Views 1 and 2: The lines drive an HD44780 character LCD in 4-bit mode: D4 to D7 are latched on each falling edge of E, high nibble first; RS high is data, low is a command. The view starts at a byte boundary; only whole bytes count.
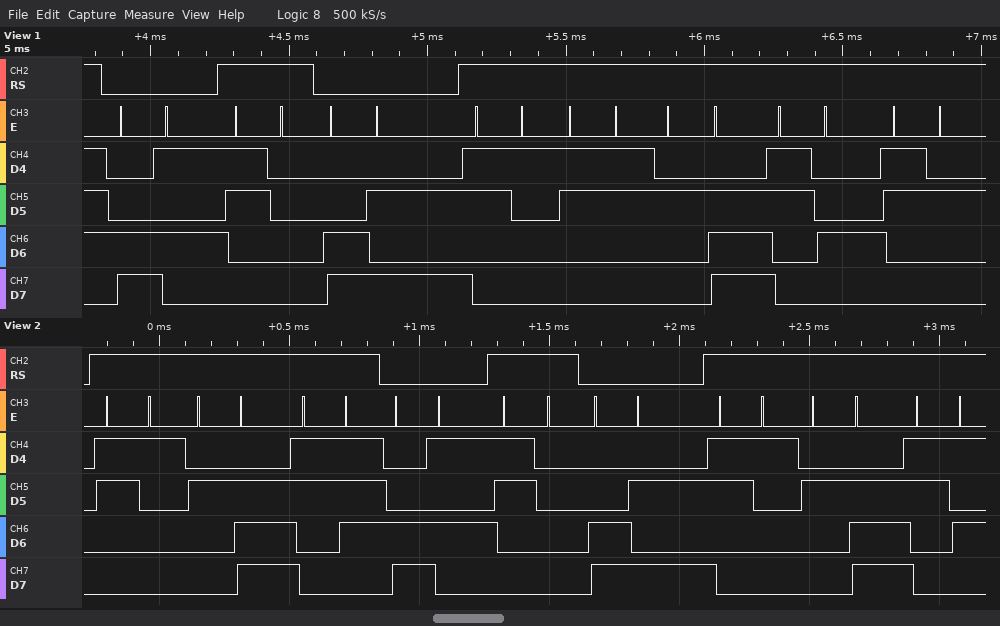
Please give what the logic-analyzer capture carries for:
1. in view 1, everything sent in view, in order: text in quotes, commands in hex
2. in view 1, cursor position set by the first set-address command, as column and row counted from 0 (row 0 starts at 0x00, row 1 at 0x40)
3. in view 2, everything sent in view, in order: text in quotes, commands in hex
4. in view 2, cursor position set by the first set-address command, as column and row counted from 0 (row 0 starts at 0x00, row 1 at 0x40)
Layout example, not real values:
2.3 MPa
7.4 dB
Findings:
0xC5 "0" 0xCA "13.42"
column 5, row 1
"1.7" 0xC5 "0" 0xCA "1.5"
column 5, row 1
